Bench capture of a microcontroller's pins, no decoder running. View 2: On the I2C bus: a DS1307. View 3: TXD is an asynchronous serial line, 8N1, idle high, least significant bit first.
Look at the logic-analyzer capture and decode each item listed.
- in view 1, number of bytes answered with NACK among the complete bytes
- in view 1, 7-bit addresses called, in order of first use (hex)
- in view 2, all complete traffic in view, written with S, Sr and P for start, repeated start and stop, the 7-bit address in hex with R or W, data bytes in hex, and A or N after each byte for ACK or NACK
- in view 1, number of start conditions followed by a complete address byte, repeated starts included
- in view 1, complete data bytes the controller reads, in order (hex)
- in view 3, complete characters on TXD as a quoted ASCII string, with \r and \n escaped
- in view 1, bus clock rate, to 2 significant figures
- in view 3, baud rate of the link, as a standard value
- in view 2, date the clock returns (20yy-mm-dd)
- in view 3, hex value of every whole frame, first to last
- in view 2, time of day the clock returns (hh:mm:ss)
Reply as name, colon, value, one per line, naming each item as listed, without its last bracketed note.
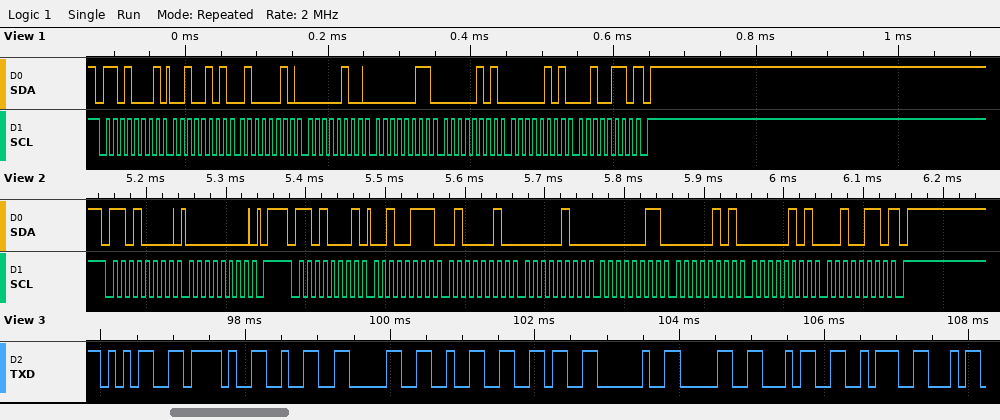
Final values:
in view 1, number of bytes answered with NACK among the complete bytes: 1
in view 1, 7-bit addresses called, in order of first use: 0x68
in view 2, all complete traffic in view, written with S, Sr and P for start, repeated start and stop, the 7-bit address in hex with R or W, data bytes in hex, and A or N after each byte for ACK or NACK: S 68W A 00 A P S 68R A 27 A 42 A 04 A 03 A 05 A 05 A 26 N P
in view 1, number of start conditions followed by a complete address byte, repeated starts included: 1
in view 1, complete data bytes the controller reads, in order: 25 42 04 03 05 05 26
in view 3, complete characters on TXD as a quoted ASCII string, with \r and \n escaped: "5/2026 04:"
in view 1, bus clock rate, to 2 significant figures: 100 kHz
in view 3, baud rate of the link, as a standard value: 9600 baud
in view 2, date the clock returns: 2026-05-05
in view 3, hex value of every whole frame, first to last: 35 2F 32 30 32 36 20 30 34 3A
in view 2, time of day the clock returns: 04:42:27
